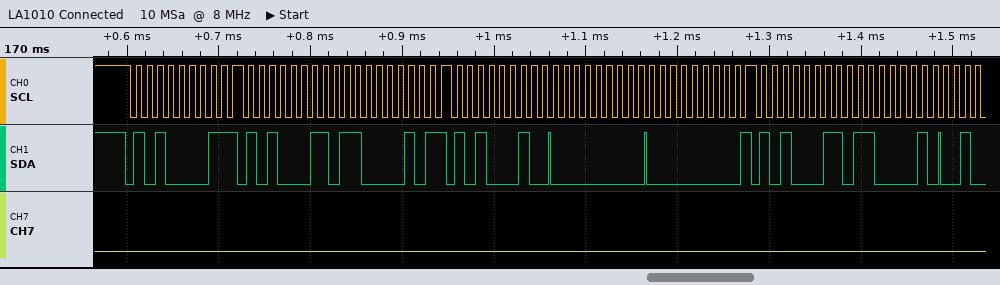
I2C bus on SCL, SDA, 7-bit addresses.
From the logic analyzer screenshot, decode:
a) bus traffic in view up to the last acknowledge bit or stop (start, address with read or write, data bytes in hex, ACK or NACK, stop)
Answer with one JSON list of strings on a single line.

["start, address 50 read NACK, repeated start, address 51 read ACK, C2 NACK, repeated start, address 51 write ACK, 00 ACK, 00 ACK, repeated start, address 51 read ACK, C2 ACK"]
